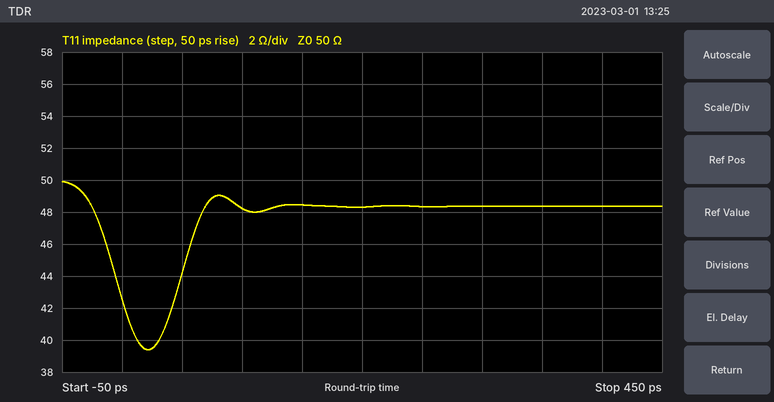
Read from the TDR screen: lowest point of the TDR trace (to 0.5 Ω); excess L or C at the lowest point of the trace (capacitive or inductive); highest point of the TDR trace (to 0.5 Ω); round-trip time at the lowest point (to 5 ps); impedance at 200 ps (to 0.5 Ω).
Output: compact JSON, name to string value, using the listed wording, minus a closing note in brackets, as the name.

{"lowest point of the TDR trace": "39.5 Ω", "excess L or C at the lowest point of the trace": "capacitive", "highest point of the TDR trace": "50.0 Ω", "round-trip time at the lowest point": "20 ps", "impedance at 200 ps": "48.5 Ω"}
